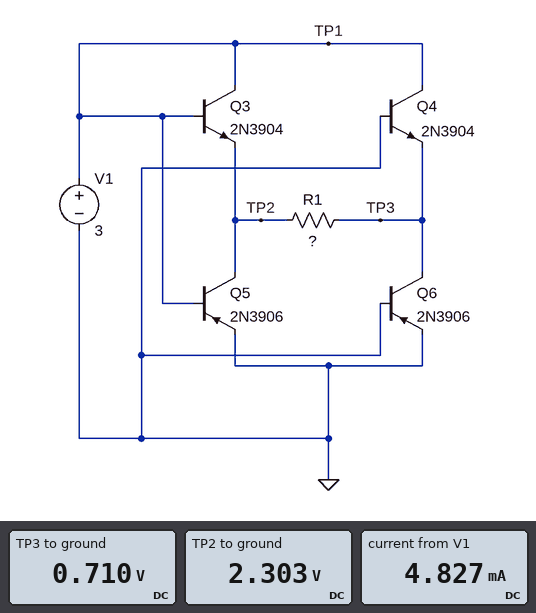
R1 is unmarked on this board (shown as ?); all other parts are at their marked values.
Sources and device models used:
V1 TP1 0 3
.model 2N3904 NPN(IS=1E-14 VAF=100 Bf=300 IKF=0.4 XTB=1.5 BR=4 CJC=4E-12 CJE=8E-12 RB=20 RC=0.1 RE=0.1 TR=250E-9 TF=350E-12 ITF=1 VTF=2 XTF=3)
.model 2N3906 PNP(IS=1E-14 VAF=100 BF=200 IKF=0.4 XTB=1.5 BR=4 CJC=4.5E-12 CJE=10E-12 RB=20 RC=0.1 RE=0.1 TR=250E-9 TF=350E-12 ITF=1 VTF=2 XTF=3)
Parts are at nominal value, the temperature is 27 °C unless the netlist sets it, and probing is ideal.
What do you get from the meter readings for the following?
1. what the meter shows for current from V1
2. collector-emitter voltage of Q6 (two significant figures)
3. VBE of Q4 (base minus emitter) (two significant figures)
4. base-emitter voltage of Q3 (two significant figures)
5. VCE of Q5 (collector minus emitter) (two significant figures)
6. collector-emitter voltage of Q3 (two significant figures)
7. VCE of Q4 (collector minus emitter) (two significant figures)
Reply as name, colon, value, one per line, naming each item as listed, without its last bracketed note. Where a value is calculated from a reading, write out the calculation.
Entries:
what the meter shows for current from V1: 4.827 mA
collector-emitter voltage of Q6: 710 mV = 710 mV
VBE of Q4 (base minus emitter): 0 V - 710 mV = -710 mV
base-emitter voltage of Q3: 3 V - 2.303 V = 700 mV
VCE of Q5 (collector minus emitter): 2.303 V = 2.3 V
collector-emitter voltage of Q3: 3 V - 2.303 V = 700 mV
VCE of Q4 (collector minus emitter): 3 V - 710 mV = 2.3 V
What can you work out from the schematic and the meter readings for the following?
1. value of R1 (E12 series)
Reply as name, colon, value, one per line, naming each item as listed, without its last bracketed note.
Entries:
value of R1: 330 Ω
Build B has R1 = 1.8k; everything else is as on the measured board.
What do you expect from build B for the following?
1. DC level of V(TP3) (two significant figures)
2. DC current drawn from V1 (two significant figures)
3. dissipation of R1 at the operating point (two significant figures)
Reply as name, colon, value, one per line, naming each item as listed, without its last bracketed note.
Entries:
DC level of V(TP3): 650 mV
DC current drawn from V1: 940 µA
dissipation of R1 at the operating point: 1.6 mW
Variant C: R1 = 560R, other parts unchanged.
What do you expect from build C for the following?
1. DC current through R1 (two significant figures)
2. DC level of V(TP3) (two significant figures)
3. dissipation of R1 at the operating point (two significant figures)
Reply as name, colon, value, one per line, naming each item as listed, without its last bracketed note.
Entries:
DC current through R1: 2.9 mA
DC level of V(TP3): 690 mV
dissipation of R1 at the operating point: 4.7 mW
